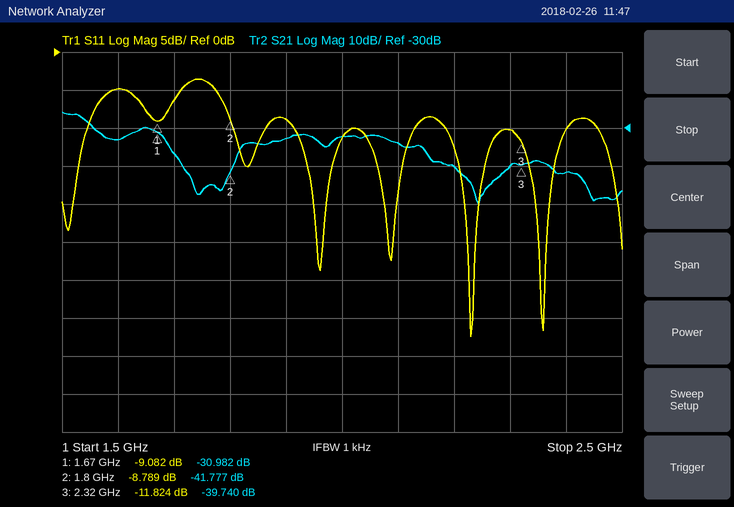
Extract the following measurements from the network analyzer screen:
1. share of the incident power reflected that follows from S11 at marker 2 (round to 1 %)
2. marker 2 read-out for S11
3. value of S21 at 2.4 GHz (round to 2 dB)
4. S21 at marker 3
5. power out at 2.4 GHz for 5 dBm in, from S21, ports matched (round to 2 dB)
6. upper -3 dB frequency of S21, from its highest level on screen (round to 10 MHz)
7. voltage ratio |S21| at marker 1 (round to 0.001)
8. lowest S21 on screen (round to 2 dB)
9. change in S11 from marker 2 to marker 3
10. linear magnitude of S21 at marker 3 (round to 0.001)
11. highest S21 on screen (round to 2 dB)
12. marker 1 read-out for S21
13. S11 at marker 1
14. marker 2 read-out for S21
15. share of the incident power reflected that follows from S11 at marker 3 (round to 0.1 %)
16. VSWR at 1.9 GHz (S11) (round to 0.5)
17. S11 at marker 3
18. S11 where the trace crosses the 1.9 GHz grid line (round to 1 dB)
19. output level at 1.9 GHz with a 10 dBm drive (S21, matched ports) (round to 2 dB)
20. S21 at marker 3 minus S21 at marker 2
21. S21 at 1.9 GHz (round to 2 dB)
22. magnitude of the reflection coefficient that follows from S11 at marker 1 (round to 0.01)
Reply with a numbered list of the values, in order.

1. 13 %
2. -8.789 dB
3. -42 dB
4. -39.740 dB
5. -36 dBm
6. 1.55 GHz
7. 0.028
8. -50 dB
9. -3.035 dB
10. 0.010
11. -26 dB
12. -30.982 dB
13. -9.082 dB
14. -41.777 dB
15. 6.6 %
16. 2.0
17. -11.824 dB
18. -9 dB
19. -22 dBm
20. 2.037 dB
21. -32 dB
22. 0.35
